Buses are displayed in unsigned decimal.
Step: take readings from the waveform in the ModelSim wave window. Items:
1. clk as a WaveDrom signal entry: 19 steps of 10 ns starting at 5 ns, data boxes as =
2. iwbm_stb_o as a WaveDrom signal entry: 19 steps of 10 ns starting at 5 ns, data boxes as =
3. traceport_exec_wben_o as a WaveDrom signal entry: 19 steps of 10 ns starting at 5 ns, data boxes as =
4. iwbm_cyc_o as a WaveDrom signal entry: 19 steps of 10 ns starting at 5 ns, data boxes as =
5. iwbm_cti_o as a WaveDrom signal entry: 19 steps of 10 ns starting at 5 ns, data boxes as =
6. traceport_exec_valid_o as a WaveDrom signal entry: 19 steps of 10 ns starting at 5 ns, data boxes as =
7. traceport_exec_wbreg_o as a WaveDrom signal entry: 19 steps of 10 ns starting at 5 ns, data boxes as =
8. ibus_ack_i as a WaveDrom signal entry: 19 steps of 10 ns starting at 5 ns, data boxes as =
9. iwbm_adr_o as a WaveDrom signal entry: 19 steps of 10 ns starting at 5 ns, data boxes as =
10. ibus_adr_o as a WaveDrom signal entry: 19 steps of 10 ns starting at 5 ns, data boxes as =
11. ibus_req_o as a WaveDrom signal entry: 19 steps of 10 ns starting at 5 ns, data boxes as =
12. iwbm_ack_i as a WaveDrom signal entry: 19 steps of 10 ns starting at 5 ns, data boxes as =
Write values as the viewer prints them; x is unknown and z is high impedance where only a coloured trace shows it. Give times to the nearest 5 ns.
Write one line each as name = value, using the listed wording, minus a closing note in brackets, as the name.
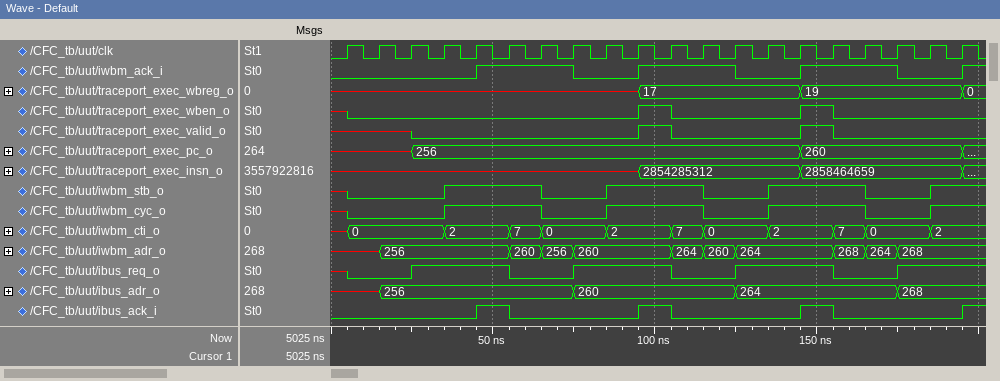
clk as a WaveDrom signal entry: 19 steps of 10 ns starting at 5 ns, data boxes as = = {name: 'clk', wave: 'p..................'}
iwbm_stb_o as a WaveDrom signal entry: 19 steps of 10 ns starting at 5 ns, data boxes as = = {name: 'iwbm_stb_o', wave: '0..1..0.1..0.1..0.1'}
traceport_exec_wben_o as a WaveDrom signal entry: 19 steps of 10 ns starting at 5 ns, data boxes as = = {name: 'traceport_exec_wben_o', wave: '0........10...10...'}
iwbm_cyc_o as a WaveDrom signal entry: 19 steps of 10 ns starting at 5 ns, data boxes as = = {name: 'iwbm_cyc_o', wave: '0..1..0.1..0.1..0.1'}
iwbm_cti_o as a WaveDrom signal entry: 19 steps of 10 ns starting at 5 ns, data boxes as = = {name: 'iwbm_cti_o', wave: '=..=.==.=.==.=.==.=', data: '0 2 7 0 2 7 0 2 7 0 2'}
traceport_exec_valid_o as a WaveDrom signal entry: 19 steps of 10 ns starting at 5 ns, data boxes as = = {name: 'traceport_exec_valid_o', wave: 'x.0......10...10...'}
traceport_exec_wbreg_o as a WaveDrom signal entry: 19 steps of 10 ns starting at 5 ns, data boxes as = = {name: 'traceport_exec_wbreg_o', wave: 'x........=....=....', data: '17 19'}
ibus_ack_i as a WaveDrom signal entry: 19 steps of 10 ns starting at 5 ns, data boxes as = = {name: 'ibus_ack_i', wave: '0...10...10...10...'}
iwbm_adr_o as a WaveDrom signal entry: 19 steps of 10 ns starting at 5 ns, data boxes as = = {name: 'iwbm_adr_o', wave: 'x=...===..===..===.', data: '256 260 256 260 264 260 264 268 264 268'}
ibus_adr_o as a WaveDrom signal entry: 19 steps of 10 ns starting at 5 ns, data boxes as = = {name: 'ibus_adr_o', wave: 'x=.....=....=....=.', data: '256 260 264 268'}
ibus_req_o as a WaveDrom signal entry: 19 steps of 10 ns starting at 5 ns, data boxes as = = {name: 'ibus_req_o', wave: '0.1..0.1..0.1..0.1.'}
iwbm_ack_i as a WaveDrom signal entry: 19 steps of 10 ns starting at 5 ns, data boxes as = = {name: 'iwbm_ack_i', wave: '0...1..0.1..0.1..0.'}
